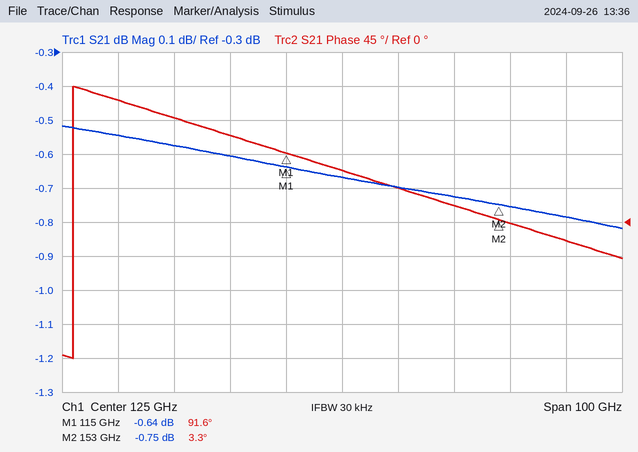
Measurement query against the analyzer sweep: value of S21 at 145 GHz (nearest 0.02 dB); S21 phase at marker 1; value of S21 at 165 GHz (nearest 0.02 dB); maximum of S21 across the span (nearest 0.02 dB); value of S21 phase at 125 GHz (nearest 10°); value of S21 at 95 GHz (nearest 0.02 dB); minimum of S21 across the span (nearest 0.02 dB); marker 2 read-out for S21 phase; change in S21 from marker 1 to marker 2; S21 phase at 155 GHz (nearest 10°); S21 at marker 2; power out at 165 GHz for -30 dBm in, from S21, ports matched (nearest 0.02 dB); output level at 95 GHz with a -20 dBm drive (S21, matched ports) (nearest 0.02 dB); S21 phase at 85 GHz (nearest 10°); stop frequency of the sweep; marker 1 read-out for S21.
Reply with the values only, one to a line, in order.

-0.72 dB
91.6°
-0.78 dB
-0.52 dB
70°
-0.58 dB
-0.82 dB
3.3°
-0.11 dB
0°
-0.75 dB
-30.78 dBm
-20.58 dBm
160°
175 GHz
-0.64 dB
